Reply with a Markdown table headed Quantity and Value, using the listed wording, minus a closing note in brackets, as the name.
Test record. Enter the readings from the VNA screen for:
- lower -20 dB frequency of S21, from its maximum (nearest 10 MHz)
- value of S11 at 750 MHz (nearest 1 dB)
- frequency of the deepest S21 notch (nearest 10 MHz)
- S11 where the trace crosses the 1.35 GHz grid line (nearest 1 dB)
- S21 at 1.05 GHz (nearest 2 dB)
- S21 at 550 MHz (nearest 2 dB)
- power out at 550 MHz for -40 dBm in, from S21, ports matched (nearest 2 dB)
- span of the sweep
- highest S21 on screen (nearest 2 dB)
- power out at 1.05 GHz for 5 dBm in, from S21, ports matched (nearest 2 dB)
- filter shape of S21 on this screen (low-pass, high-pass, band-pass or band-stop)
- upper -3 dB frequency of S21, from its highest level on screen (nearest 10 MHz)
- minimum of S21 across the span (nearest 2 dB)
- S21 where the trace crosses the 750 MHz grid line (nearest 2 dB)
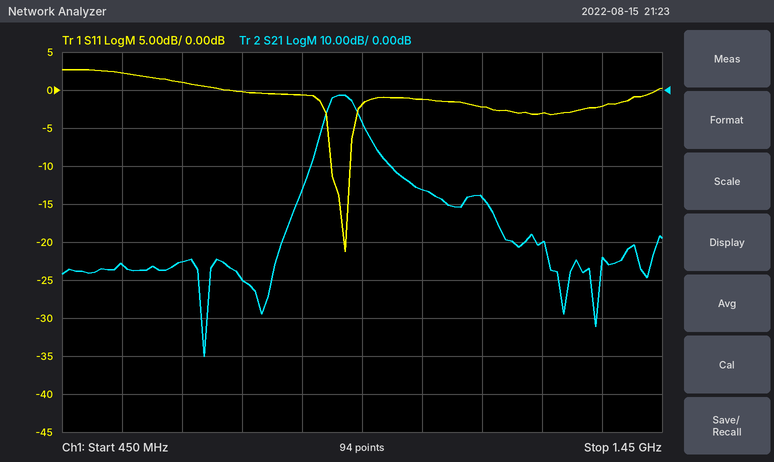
| Quantity | Value |
|---|---|
| lower -20 dB frequency of S21, from its maximum | 860 MHz |
| value of S11 at 750 MHz | 0 dB |
| frequency of the deepest S21 notch | 690 MHz |
| S11 where the trace crosses the 1.35 GHz grid line | -2 dB |
| S21 at 1.05 GHz | -26 dB |
| S21 at 550 MHz | -46 dB |
| power out at 550 MHz for -40 dBm in, from S21, ports matched | -86 dBm |
| span of the sweep | 1 GHz |
| highest S21 on screen | -2 dB |
| power out at 1.05 GHz for 5 dBm in, from S21, ports matched | -22 dBm |
| filter shape of S21 on this screen | band-pass |
| upper -3 dB frequency of S21, from its highest level on screen | 940 MHz |
| minimum of S21 across the span | -70 dB |
| S21 where the trace crosses the 750 MHz grid line | -50 dB |
